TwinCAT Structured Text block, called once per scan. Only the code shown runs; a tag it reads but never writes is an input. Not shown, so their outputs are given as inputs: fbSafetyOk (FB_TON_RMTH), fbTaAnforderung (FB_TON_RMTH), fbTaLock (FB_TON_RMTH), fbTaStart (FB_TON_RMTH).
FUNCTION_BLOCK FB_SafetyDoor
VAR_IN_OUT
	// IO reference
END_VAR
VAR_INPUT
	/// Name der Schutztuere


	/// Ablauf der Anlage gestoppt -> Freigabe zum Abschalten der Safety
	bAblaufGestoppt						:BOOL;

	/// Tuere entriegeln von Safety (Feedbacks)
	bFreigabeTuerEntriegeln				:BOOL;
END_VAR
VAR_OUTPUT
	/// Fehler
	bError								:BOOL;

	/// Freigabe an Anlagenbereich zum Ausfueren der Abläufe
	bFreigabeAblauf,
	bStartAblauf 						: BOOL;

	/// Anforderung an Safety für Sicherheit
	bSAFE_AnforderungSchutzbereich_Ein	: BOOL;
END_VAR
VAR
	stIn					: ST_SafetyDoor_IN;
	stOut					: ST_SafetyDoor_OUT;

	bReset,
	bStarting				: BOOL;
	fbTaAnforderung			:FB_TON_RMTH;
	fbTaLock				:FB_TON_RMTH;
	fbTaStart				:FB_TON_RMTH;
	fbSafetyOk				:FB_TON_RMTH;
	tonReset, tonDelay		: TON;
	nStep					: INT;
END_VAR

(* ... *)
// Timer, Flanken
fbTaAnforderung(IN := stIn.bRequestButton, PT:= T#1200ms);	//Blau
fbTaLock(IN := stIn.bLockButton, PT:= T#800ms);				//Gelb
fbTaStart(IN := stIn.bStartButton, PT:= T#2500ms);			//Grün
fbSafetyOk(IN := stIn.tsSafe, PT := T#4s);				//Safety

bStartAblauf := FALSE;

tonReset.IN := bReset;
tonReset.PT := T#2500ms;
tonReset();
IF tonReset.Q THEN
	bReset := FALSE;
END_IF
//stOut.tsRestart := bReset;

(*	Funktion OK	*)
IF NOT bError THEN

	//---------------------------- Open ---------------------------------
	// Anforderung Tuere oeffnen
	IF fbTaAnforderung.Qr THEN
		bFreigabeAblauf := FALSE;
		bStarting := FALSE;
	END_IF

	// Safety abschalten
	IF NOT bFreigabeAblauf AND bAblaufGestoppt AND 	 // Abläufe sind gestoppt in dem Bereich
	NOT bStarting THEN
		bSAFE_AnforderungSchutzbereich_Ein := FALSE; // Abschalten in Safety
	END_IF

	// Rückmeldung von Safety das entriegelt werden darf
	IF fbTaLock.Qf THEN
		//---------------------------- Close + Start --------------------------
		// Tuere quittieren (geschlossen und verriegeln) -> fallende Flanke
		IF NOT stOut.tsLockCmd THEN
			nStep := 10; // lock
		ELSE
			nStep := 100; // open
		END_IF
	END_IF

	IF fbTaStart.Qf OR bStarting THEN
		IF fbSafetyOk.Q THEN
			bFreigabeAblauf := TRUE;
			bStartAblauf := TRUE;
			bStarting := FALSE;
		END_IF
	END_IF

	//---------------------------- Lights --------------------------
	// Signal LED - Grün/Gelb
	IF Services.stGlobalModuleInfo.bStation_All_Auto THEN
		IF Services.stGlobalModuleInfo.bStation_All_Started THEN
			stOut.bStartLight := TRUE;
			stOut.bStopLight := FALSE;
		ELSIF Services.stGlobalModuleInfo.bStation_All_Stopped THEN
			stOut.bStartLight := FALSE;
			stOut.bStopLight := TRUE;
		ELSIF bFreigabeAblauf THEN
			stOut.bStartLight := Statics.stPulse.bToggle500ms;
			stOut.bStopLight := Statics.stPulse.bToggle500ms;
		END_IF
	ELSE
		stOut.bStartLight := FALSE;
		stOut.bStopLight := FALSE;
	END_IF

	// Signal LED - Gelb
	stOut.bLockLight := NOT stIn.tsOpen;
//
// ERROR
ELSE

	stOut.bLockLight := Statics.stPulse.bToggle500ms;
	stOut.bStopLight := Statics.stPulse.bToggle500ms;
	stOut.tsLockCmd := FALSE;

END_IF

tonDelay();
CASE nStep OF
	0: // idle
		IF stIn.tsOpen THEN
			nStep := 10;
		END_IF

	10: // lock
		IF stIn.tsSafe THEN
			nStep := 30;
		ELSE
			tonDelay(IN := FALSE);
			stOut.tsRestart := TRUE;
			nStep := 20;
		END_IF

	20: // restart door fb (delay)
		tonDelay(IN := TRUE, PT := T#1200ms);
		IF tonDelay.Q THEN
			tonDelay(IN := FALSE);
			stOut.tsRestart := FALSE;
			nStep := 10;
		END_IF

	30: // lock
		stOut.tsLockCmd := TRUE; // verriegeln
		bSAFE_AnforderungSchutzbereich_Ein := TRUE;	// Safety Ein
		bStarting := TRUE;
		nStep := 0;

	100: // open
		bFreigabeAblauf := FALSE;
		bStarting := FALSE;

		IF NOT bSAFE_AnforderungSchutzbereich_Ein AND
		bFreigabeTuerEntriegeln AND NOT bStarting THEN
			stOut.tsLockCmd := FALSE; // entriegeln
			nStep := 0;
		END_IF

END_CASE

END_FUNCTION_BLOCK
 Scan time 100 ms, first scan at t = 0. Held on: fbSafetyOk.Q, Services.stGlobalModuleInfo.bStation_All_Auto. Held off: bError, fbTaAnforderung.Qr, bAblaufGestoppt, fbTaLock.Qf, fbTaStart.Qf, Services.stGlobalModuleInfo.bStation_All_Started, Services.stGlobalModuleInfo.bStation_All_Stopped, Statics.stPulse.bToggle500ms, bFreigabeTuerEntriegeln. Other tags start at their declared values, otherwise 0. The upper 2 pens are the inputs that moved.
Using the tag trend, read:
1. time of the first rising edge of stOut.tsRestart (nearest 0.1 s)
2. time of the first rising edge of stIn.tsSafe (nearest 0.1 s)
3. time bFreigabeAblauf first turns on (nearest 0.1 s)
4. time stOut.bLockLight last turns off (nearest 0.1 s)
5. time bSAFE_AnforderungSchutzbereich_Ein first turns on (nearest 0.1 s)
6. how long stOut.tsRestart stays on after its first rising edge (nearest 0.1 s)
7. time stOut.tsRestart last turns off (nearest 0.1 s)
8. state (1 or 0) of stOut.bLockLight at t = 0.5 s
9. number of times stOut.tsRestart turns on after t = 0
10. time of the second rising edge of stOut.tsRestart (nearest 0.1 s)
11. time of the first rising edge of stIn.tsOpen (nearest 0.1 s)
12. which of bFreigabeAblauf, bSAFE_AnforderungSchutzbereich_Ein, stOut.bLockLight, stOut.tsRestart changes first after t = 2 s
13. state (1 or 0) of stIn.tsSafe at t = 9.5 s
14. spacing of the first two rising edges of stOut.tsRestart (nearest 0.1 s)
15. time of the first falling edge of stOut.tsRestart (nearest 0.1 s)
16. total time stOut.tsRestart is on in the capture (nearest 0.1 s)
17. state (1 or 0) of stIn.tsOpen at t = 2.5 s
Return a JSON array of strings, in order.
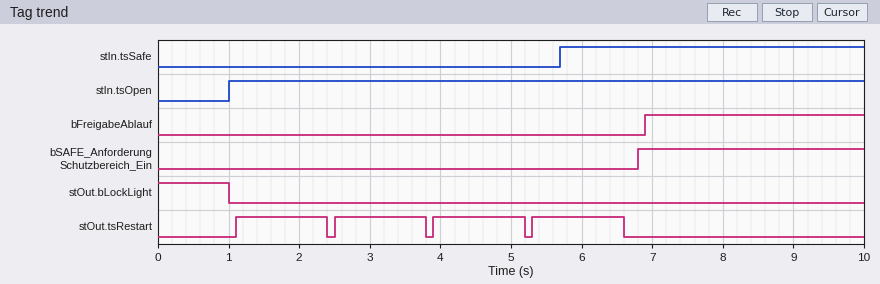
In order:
["1.1 s", "5.7 s", "6.9 s", "1.0 s", "6.8 s", "1.3 s", "6.6 s", "1", "4", "2.5 s", "1.0 s", "stOut.tsRestart", "1", "1.4 s", "2.4 s", "5.2 s", "1"]
